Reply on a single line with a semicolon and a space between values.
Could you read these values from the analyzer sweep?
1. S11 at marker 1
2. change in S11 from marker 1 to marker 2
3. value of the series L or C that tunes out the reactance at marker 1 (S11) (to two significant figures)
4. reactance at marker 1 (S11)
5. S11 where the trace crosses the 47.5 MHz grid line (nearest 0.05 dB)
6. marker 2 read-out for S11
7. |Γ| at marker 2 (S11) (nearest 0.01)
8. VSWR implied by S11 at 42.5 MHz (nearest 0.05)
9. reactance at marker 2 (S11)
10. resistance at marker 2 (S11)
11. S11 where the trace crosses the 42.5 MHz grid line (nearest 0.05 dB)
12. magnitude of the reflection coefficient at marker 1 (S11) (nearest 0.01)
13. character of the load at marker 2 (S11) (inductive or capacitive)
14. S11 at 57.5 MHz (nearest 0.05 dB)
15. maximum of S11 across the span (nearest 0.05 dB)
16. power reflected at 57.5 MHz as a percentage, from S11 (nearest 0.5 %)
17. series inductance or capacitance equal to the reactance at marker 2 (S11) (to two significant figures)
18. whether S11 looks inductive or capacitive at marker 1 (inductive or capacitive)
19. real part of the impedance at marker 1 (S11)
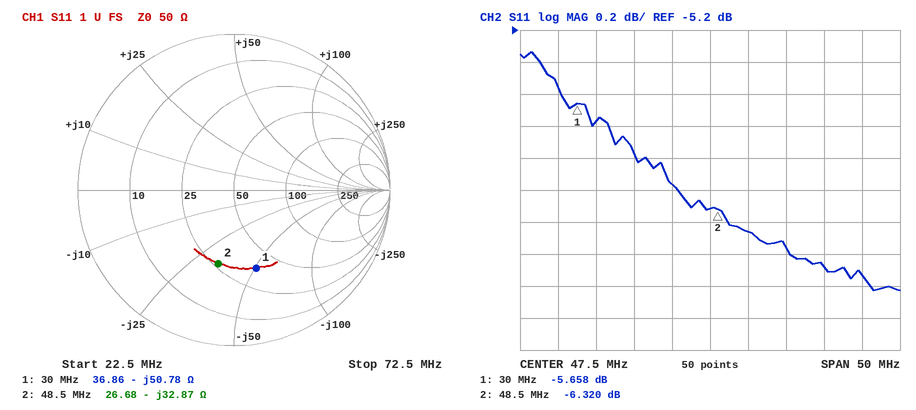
-5.658 dB; -0.662 dB; 270 nH; -50.78 Ω; -6.30 dB; -6.320 dB; 0.48; 2.95; -32.87 Ω; 26.68 Ω; -6.15 dB; 0.52; capacitive; -6.55 dB; -5.35 dB; 22.0 %; 100 pF; capacitive; 36.86 Ω
